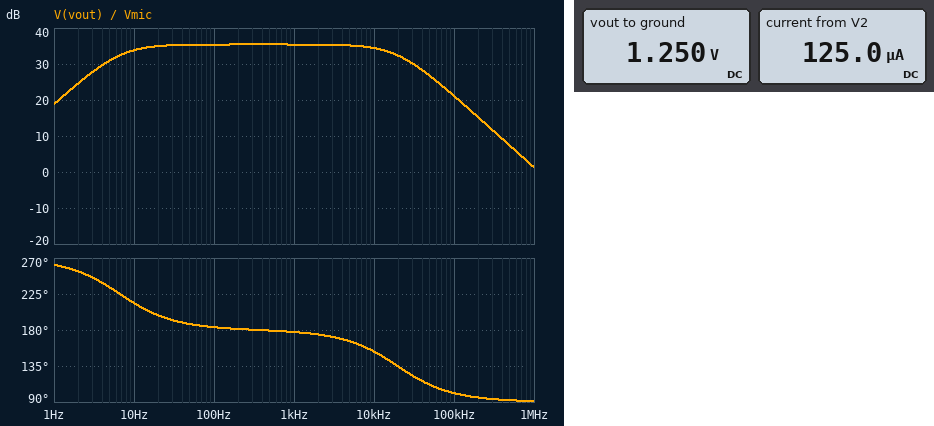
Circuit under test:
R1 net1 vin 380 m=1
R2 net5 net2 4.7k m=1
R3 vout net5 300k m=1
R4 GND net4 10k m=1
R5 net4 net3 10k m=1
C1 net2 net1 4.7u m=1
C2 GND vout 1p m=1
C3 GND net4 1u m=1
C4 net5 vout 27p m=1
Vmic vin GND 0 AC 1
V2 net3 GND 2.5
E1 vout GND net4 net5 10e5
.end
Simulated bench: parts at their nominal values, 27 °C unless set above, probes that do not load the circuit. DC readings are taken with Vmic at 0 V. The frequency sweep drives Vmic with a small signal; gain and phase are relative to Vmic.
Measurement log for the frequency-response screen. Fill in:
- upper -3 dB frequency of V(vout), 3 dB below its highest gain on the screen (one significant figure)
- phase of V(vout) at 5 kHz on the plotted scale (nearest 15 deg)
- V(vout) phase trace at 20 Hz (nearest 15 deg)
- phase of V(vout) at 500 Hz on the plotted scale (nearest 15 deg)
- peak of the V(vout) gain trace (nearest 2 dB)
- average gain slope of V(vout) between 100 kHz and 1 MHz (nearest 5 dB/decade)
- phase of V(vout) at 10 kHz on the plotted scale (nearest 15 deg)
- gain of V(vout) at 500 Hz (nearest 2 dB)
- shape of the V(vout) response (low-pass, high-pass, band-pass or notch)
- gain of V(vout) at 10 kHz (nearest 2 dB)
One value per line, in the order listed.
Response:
20 kHz
165 deg
195 deg
180 deg
36 dB
-20 dB/decade
150 deg
36 dB
band-pass
34 dB
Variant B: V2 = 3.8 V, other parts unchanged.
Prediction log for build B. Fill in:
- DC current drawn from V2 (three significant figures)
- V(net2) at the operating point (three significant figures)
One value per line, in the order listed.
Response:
190 µA
1.90 V
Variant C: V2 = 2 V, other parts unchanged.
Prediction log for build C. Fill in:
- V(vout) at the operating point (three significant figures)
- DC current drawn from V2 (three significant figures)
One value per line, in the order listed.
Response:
1.00 V
100 µA
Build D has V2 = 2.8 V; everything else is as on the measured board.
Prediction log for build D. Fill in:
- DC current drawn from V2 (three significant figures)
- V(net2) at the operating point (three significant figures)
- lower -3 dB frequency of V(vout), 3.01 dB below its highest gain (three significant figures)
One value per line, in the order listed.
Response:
140 µA
1.40 V
6.66 Hz
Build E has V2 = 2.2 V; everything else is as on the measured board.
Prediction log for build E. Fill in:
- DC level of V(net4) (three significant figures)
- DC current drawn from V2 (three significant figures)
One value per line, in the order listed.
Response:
1.10 V
110 µA
